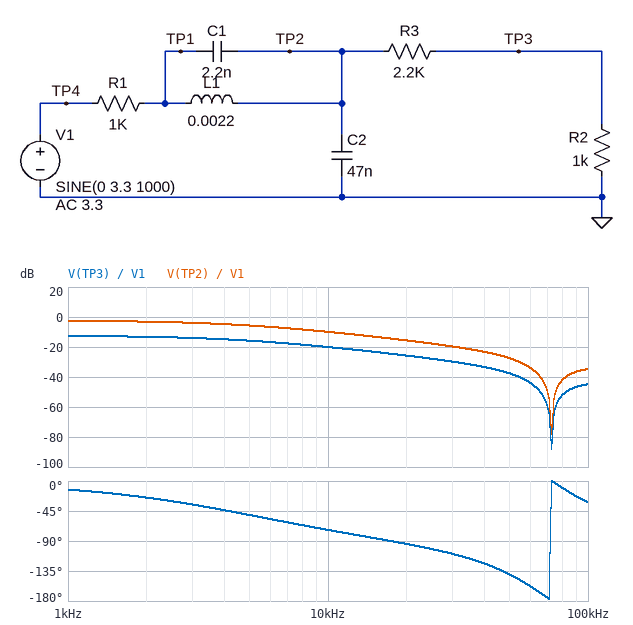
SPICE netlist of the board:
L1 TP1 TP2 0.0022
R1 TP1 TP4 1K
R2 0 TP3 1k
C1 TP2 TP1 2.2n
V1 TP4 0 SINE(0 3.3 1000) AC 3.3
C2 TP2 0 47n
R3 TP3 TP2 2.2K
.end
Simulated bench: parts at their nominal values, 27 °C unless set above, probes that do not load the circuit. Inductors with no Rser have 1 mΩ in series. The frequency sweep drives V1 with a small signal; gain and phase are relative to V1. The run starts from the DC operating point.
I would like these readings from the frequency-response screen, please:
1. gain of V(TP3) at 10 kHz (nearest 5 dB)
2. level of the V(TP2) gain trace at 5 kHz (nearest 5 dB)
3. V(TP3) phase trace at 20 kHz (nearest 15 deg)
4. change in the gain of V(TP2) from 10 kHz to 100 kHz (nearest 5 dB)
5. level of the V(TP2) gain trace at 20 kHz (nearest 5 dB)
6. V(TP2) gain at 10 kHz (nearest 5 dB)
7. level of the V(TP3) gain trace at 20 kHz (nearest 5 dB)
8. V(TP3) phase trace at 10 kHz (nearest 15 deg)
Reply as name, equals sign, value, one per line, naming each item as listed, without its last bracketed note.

gain of V(TP3) at 10 kHz = -20 dB
level of the V(TP2) gain trace at 5 kHz = -5 dB
V(TP3) phase trace at 20 kHz = -90 deg
change in the gain of V(TP2) from 10 kHz to 100 kHz = -25 dB
level of the V(TP2) gain trace at 20 kHz = -15 dB
V(TP2) gain at 10 kHz = -10 dB
level of the V(TP3) gain trace at 20 kHz = -25 dB
V(TP3) phase trace at 10 kHz = -75 deg
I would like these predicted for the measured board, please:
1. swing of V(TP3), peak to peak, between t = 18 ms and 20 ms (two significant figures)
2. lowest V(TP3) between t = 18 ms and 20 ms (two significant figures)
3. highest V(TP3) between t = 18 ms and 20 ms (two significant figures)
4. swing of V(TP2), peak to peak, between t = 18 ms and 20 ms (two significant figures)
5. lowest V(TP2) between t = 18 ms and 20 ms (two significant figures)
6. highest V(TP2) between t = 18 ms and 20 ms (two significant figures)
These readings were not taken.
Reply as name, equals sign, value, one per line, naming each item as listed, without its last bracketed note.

swing of V(TP3), peak to peak, between t = 18 ms and 20 ms = 1.5 V
lowest V(TP3) between t = 18 ms and 20 ms = -770 mV
highest V(TP3) between t = 18 ms and 20 ms = 770 mV
swing of V(TP2), peak to peak, between t = 18 ms and 20 ms = 4.9 V
lowest V(TP2) between t = 18 ms and 20 ms = -2.5 V
highest V(TP2) between t = 18 ms and 20 ms = 2.5 V
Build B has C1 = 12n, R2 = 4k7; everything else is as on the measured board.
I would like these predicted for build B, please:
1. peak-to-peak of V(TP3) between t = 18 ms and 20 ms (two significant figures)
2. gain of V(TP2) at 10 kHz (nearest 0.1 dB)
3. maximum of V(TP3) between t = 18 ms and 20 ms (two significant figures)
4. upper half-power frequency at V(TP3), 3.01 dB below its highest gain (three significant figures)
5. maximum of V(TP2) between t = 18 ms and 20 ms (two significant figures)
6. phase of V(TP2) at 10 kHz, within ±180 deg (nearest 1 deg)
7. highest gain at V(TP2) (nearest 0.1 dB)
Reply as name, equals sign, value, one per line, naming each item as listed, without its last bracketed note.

peak-to-peak of V(TP3) between t = 18 ms and 20 ms = 3.8 V
gain of V(TP2) at 10 kHz = -9.7 dB
maximum of V(TP3) between t = 18 ms and 20 ms = 1.9 V
upper half-power frequency at V(TP3), 3.01 dB below its highest gain = 4.07 kHz
maximum of V(TP2) between t = 18 ms and 20 ms = 2.8 V
phase of V(TP2) at 10 kHz, within ±180 deg = -77 deg
highest gain at V(TP2) = -1.2 dB
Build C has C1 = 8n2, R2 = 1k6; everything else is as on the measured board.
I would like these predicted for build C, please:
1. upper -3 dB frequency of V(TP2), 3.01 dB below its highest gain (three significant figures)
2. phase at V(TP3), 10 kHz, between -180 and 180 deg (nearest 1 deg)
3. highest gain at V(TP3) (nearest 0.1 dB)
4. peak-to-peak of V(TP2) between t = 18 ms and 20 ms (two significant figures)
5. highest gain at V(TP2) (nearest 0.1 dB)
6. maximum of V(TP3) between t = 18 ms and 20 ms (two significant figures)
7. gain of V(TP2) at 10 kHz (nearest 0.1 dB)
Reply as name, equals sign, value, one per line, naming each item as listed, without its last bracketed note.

upper -3 dB frequency of V(TP2), 3.01 dB below its highest gain = 4.49 kHz
phase at V(TP3), 10 kHz, between -180 and 180 deg = -75 deg
highest gain at V(TP3) = -9.5 dB
peak-to-peak of V(TP2) between t = 18 ms and 20 ms = 5.1 V
highest gain at V(TP2) = -2.0 dB
maximum of V(TP3) between t = 18 ms and 20 ms = 1.1 V
gain of V(TP2) at 10 kHz = -9.8 dB
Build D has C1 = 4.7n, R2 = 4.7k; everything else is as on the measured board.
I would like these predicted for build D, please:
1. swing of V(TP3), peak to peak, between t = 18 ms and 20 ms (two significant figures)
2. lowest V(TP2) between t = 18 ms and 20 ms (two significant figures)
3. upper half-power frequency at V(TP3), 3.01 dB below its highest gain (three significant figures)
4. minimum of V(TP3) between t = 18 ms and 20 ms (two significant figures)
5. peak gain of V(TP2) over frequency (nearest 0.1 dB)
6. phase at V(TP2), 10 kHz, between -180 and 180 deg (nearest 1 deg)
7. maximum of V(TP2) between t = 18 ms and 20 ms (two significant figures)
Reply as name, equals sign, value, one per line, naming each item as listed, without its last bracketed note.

swing of V(TP3), peak to peak, between t = 18 ms and 20 ms = 3.8 V
lowest V(TP2) between t = 18 ms and 20 ms = -2.8 V
upper half-power frequency at V(TP3), 3.01 dB below its highest gain = 4.07 kHz
minimum of V(TP3) between t = 18 ms and 20 ms = -1.9 V
peak gain of V(TP2) over frequency = -1.2 dB
phase at V(TP2), 10 kHz, between -180 and 180 deg = -76 deg
maximum of V(TP2) between t = 18 ms and 20 ms = 2.8 V
